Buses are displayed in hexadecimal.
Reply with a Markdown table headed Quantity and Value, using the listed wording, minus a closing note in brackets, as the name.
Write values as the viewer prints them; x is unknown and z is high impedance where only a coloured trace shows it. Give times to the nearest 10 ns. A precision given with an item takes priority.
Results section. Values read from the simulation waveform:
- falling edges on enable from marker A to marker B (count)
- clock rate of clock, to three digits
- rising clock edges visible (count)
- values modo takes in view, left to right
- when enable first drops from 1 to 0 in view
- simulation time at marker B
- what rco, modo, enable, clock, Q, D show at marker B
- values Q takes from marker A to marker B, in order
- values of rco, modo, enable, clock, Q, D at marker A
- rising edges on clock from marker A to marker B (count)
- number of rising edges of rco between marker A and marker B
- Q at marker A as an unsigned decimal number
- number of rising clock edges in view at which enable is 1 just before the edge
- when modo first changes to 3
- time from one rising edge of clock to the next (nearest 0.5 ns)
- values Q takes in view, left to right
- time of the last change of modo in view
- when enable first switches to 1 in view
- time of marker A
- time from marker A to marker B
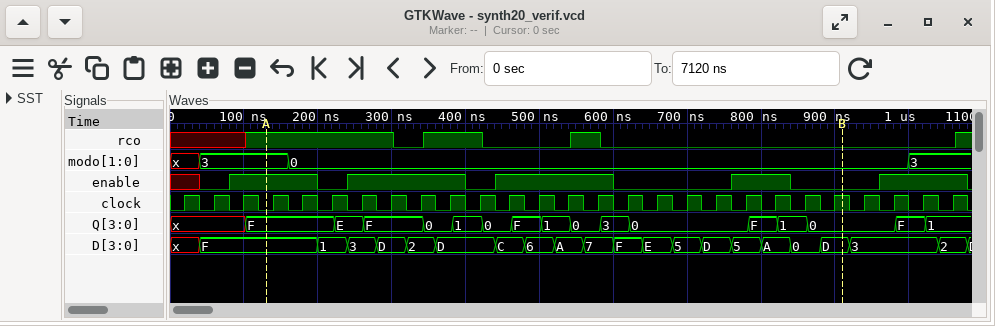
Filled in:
| Quantity | Value |
|---|---|
| falling edges on enable from marker A to marker B | 4 |
| clock rate of clock, to three digits | 25.0 MHz |
| rising clock edges visible | 27 |
| values modo takes in view, left to right | x, 3, 0, 3 |
| when enable first drops from 1 to 0 in view | 200 ns |
| simulation time at marker B | 910 ns |
| what rco, modo, enable, clock, Q, D show at marker B | rco=0, modo=0, enable=0, clock=1, Q=0, D=D |
| values Q takes from marker A to marker B, in order | F, E, F, 0, 1, 0, F, 1, 0, 3, 0, F, 1, 0 |
| values of rco, modo, enable, clock, Q, D at marker A | rco=1, modo=3, enable=1, clock=0, Q=F, D=F |
| rising edges on clock from marker A to marker B | 20 |
| number of rising edges of rco between marker A and marker B | 2 |
| Q at marker A as an unsigned decimal number | 15 |
| number of rising clock edges in view at which enable is 1 just before the edge | 16 |
| when modo first changes to 3 | 40 ns |
| time from one rising edge of clock to the next | 40 ns |
| values Q takes in view, left to right | x, F, E, F, 0, 1, 0, F, 1, 0, 3, 0, F, 1, 0, F, 1 |
| time of the last change of modo in view | 1000 ns |
| when enable first switches to 1 in view | 80 ns |
| time of marker A | 130 ns |
| time from marker A to marker B | 780 ns |
